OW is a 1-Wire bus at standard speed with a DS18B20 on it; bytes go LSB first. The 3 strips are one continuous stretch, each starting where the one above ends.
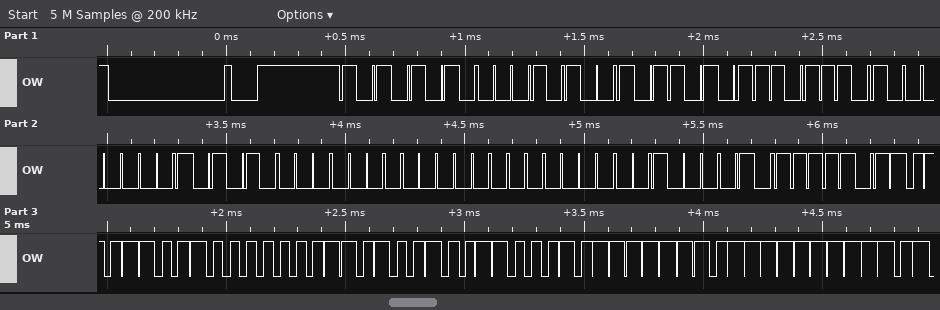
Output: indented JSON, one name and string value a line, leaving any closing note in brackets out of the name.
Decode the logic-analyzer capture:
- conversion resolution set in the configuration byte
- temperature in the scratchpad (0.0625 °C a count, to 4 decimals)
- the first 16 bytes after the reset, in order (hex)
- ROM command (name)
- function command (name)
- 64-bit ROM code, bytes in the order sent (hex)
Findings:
{
  "conversion resolution set in the configuration byte": "12 bits",
  "temperature in the scratchpad": "19.3125 °C",
  "the first 16 bytes after the reset, in order": "55 28 AD BB 80 0A 00 00 84 BE 35 01 4B 46 7F FF",
  "ROM command": "Match ROM",
  "function command": "Read Scratchpad",
  "64-bit ROM code, bytes in the order sent": "28 AD BB 80 0A 00 00 84"
}
